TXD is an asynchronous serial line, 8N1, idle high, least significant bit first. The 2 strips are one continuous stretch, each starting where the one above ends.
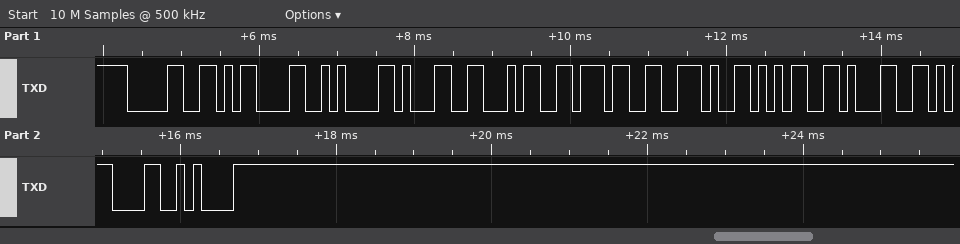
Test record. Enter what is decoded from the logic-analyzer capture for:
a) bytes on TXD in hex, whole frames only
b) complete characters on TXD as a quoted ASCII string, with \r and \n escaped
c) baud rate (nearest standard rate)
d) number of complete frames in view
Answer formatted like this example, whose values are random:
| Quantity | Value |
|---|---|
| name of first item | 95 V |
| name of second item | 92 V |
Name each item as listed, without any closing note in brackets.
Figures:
| Quantity | Value |
|---|---|
| bytes on TXD in hex, whole frames only | 30 0D 0A 31 34 37 2E 35 31 0D 0A |
| complete characters on TXD as a quoted ASCII string, with \r and \n escaped | "0\r\n147.51\r\n" |
| baud rate | 9600 baud |
| number of complete frames in view | 11 |
